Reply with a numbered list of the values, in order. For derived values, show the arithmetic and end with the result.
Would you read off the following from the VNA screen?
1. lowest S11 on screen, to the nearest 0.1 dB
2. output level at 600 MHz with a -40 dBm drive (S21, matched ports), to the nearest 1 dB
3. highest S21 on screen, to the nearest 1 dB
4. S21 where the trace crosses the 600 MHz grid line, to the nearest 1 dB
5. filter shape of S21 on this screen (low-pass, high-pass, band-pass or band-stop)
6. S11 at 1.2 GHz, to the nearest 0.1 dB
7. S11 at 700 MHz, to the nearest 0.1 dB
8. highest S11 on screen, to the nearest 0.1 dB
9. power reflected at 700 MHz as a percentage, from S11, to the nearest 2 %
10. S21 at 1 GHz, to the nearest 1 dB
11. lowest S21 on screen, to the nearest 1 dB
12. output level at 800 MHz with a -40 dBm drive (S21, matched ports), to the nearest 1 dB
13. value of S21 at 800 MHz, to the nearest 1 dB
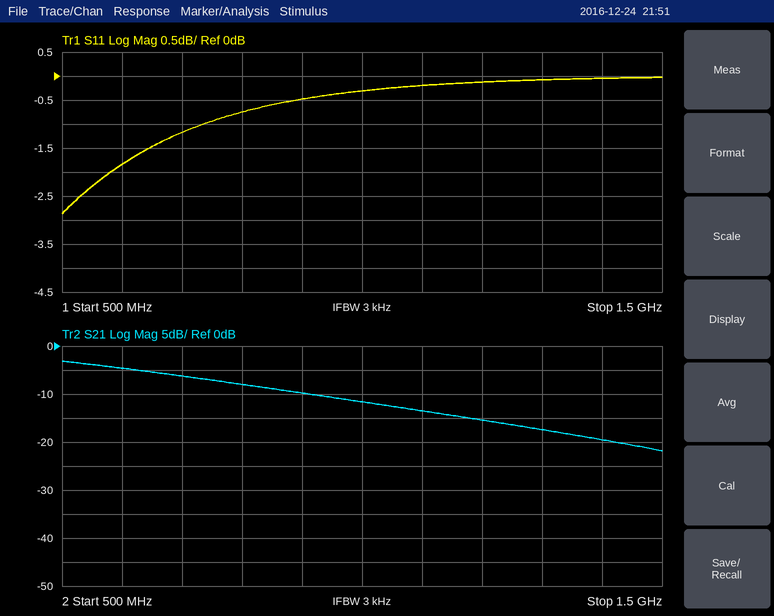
1. -2.9 dB
2. -40 dBm + (-5 dB) = -45 dBm
3. -3 dB
4. -5 dB
5. low-pass
6. -0.1 dB
7. -1.2 dB
8. 0.0 dB
9. 10^(-1.2/10) ≈ 76 %
10. -12 dB
11. -22 dB
12. -40 dBm + (-8 dB) = -48 dBm
13. -8 dB
